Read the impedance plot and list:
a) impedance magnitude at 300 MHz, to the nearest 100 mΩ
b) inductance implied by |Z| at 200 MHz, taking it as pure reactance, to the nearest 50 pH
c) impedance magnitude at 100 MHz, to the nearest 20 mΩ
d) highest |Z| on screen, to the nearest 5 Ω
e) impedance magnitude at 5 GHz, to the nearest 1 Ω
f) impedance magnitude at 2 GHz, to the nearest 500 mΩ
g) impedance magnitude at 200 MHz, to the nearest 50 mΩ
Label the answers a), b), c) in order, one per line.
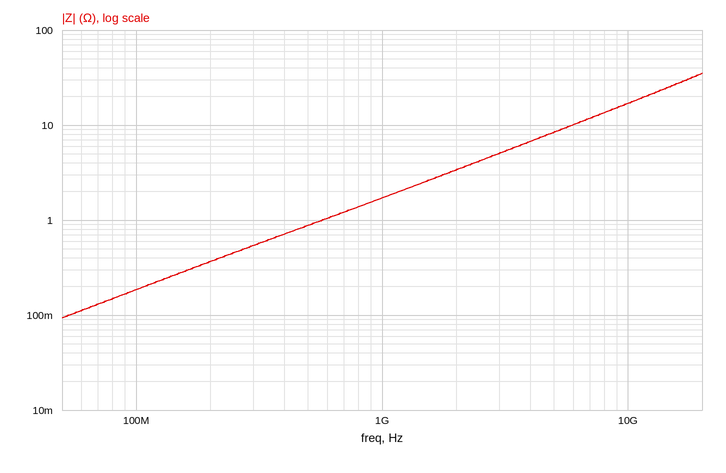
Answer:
a) 500 mΩ
b) 300 pH
c) 180 mΩ
d) 35 Ω
e) 8 Ω
f) 3.5 Ω
g) 350 mΩ
